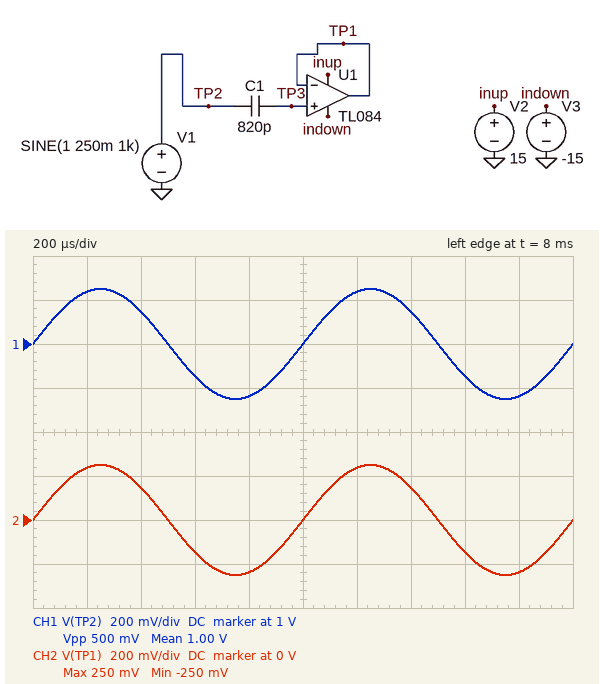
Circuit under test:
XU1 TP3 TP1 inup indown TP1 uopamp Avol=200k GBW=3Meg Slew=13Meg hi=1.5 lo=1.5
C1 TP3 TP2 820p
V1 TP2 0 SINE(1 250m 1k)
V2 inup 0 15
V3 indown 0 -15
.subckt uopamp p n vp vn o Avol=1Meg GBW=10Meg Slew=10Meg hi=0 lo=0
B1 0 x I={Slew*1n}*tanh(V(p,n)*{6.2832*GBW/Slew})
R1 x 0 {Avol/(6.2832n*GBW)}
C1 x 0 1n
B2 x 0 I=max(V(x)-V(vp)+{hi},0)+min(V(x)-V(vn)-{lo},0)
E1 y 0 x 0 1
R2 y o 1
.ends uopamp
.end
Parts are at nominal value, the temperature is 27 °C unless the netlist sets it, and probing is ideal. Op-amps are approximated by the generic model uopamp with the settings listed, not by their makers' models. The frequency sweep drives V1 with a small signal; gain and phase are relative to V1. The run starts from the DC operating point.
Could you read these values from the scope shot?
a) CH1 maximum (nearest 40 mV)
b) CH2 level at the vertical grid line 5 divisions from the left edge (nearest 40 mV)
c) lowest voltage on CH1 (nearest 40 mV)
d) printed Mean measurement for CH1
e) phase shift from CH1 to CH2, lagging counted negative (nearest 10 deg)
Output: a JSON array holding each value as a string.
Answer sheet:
["1.24 V", "0 V", "760 mV", "1.00 V", "0 deg"]
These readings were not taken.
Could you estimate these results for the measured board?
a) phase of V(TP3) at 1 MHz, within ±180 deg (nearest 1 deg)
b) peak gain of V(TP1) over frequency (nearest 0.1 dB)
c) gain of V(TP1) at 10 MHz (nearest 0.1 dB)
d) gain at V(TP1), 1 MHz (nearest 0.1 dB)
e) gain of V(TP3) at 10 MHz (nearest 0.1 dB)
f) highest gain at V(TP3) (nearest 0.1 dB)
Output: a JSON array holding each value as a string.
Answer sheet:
["0 deg", "0 dB", "-10.8 dB", "-0.5 dB", "0 dB", "0 dB"]
